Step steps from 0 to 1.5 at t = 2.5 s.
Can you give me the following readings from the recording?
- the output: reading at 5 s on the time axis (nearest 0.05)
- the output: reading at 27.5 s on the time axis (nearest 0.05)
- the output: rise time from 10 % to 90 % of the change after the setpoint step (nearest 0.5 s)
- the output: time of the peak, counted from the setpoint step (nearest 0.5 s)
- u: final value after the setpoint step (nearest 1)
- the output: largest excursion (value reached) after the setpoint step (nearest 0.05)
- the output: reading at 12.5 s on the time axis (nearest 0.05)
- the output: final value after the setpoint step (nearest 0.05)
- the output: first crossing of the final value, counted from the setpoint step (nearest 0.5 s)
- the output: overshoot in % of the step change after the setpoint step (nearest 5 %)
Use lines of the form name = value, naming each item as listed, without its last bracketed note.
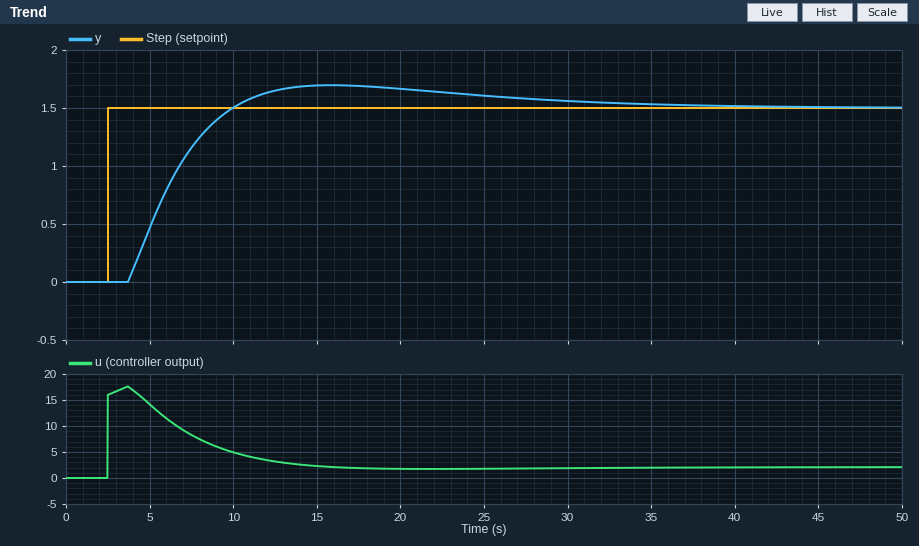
the output: reading at 5 s on the time axis = 0.45
the output: reading at 27.5 s on the time axis = 1.60
the output: rise time from 10 % to 90 % of the change after the setpoint step = 4.5 s
the output: time of the peak, counted from the setpoint step = 13.5 s
u: final value after the setpoint step = 2
the output: largest excursion (value reached) after the setpoint step = 1.70
the output: reading at 12.5 s on the time axis = 1.65
the output: final value after the setpoint step = 1.50
the output: first crossing of the final value, counted from the setpoint step = 7.5 s
the output: overshoot in % of the step change after the setpoint step = 15 %
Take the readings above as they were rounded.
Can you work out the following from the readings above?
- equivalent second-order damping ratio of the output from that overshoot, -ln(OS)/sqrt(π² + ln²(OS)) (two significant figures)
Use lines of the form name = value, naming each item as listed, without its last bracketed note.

equivalent second-order damping ratio of the output from that overshoot, -ln(OS)/sqrt(π² + ln²(OS)) = 0.52
